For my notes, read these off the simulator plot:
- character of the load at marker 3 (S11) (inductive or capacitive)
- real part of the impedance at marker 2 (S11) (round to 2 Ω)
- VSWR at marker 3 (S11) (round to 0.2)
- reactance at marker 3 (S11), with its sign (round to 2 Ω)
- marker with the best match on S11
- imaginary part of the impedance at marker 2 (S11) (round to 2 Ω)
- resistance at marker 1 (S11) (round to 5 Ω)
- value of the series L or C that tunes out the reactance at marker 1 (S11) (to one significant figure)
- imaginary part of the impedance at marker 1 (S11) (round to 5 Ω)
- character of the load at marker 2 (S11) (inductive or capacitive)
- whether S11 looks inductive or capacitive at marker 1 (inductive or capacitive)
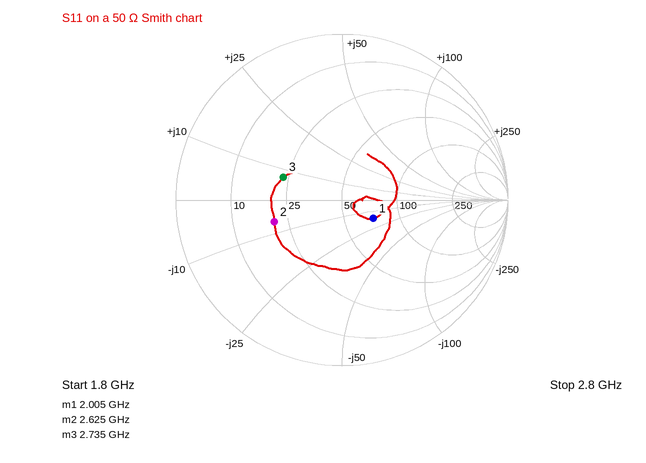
inductive
20 Ω
2.2
+8 Ω
marker 1
-6 Ω
70 Ω
1 nH
-15 Ω
capacitive
capacitive
